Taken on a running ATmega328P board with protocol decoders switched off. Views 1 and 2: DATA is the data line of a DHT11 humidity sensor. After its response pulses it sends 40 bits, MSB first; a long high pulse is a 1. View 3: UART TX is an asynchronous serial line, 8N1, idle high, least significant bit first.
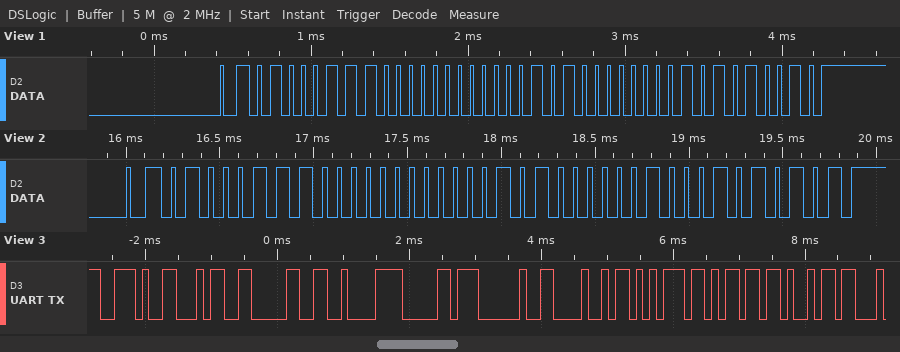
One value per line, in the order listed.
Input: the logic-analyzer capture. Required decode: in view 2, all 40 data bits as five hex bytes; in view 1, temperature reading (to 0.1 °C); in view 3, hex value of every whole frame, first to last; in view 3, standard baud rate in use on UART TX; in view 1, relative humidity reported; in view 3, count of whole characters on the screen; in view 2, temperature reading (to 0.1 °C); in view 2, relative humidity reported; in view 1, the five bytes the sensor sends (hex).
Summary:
47 00 0A 04 55
10.1 °C
2E 34 30 C2 B0 20 48 75 6D 69
9600 baud
71 %
10
10.4 °C
71 %
47 00 0A 01 52
